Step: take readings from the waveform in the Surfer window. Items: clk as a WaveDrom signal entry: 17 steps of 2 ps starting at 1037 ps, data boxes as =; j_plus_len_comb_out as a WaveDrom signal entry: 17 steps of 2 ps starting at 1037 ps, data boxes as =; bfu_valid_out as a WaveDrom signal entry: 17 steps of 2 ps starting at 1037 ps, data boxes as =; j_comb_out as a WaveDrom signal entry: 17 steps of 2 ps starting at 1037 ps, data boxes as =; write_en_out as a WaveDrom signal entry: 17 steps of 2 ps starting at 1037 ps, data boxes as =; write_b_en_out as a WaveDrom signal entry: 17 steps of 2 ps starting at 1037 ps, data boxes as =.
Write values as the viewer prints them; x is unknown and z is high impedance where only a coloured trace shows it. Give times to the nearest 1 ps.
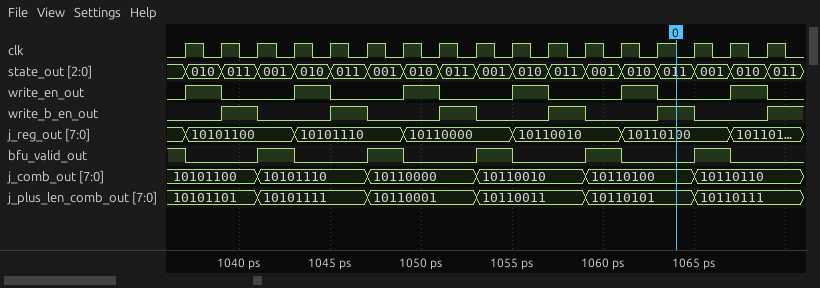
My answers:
{name: 'clk', wave: 'p................'}
{name: 'j_plus_len_comb_out', wave: '=.=..=..=..=..=..', data: '10101101 10101111 10110001 10110011 10110101 10110111'}
{name: 'bfu_valid_out', wave: '0.10.10.10.10.10.'}
{name: 'j_comb_out', wave: '=.=..=..=..=..=..', data: '10101100 10101110 10110000 10110010 10110100 10110110'}
{name: 'write_en_out', wave: '10.10.10.10.10.10'}
{name: 'write_b_en_out', wave: '010.10.10.10.10.1'}
